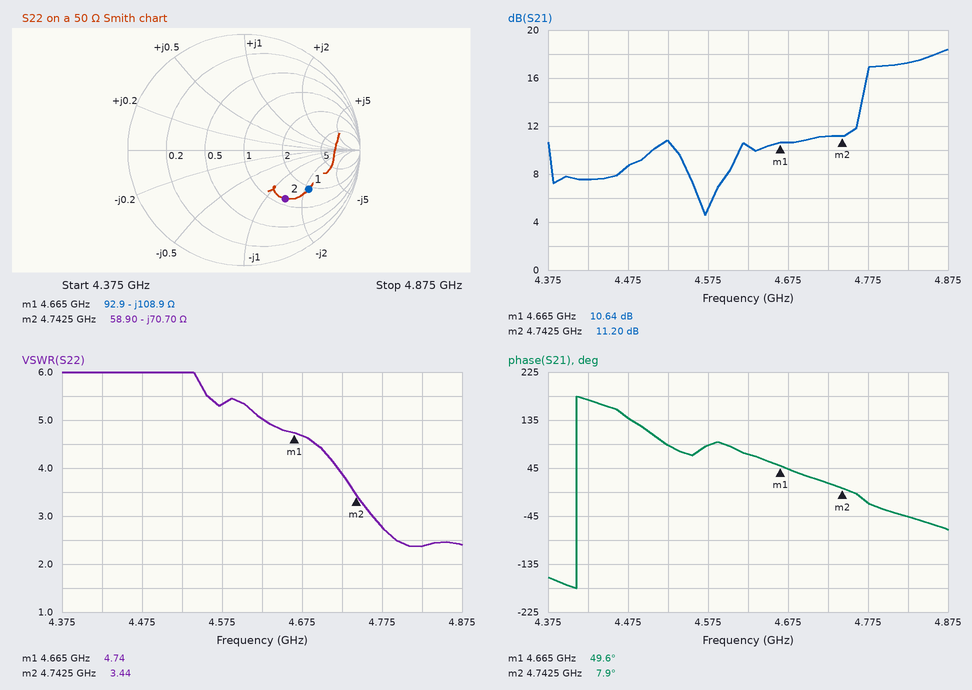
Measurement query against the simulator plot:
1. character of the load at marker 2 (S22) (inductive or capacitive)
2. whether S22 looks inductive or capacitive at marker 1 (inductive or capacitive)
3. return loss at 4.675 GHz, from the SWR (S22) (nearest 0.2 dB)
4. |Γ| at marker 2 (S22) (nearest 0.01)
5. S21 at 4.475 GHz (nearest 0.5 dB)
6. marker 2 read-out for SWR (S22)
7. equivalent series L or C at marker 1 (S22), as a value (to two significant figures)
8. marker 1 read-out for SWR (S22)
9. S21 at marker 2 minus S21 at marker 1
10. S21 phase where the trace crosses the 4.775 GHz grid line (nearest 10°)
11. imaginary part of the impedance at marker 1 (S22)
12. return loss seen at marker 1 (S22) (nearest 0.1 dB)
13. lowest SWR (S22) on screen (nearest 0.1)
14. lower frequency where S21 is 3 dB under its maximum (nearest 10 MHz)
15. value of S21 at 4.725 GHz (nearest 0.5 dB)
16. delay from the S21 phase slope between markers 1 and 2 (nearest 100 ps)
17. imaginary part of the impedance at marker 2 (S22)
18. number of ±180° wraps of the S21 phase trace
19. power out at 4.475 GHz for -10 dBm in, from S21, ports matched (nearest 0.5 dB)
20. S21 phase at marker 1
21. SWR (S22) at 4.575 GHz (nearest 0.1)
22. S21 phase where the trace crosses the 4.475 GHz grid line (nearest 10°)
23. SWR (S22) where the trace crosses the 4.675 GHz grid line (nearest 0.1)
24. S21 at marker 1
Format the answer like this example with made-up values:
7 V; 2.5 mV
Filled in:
capacitive; capacitive; 3.8 dB; 0.55; 8.5 dB; 3.44; 310 fF; 4.74; 0.56 dB; -20°; -108.9 Ω; 3.7 dB; 2.4; 4.77 GHz; 11.0 dB; 1.5 ns; -70.70 Ω; 1; -1.5 dBm; 49.6°; 5.3; 140°; 4.7; 10.64 dB
